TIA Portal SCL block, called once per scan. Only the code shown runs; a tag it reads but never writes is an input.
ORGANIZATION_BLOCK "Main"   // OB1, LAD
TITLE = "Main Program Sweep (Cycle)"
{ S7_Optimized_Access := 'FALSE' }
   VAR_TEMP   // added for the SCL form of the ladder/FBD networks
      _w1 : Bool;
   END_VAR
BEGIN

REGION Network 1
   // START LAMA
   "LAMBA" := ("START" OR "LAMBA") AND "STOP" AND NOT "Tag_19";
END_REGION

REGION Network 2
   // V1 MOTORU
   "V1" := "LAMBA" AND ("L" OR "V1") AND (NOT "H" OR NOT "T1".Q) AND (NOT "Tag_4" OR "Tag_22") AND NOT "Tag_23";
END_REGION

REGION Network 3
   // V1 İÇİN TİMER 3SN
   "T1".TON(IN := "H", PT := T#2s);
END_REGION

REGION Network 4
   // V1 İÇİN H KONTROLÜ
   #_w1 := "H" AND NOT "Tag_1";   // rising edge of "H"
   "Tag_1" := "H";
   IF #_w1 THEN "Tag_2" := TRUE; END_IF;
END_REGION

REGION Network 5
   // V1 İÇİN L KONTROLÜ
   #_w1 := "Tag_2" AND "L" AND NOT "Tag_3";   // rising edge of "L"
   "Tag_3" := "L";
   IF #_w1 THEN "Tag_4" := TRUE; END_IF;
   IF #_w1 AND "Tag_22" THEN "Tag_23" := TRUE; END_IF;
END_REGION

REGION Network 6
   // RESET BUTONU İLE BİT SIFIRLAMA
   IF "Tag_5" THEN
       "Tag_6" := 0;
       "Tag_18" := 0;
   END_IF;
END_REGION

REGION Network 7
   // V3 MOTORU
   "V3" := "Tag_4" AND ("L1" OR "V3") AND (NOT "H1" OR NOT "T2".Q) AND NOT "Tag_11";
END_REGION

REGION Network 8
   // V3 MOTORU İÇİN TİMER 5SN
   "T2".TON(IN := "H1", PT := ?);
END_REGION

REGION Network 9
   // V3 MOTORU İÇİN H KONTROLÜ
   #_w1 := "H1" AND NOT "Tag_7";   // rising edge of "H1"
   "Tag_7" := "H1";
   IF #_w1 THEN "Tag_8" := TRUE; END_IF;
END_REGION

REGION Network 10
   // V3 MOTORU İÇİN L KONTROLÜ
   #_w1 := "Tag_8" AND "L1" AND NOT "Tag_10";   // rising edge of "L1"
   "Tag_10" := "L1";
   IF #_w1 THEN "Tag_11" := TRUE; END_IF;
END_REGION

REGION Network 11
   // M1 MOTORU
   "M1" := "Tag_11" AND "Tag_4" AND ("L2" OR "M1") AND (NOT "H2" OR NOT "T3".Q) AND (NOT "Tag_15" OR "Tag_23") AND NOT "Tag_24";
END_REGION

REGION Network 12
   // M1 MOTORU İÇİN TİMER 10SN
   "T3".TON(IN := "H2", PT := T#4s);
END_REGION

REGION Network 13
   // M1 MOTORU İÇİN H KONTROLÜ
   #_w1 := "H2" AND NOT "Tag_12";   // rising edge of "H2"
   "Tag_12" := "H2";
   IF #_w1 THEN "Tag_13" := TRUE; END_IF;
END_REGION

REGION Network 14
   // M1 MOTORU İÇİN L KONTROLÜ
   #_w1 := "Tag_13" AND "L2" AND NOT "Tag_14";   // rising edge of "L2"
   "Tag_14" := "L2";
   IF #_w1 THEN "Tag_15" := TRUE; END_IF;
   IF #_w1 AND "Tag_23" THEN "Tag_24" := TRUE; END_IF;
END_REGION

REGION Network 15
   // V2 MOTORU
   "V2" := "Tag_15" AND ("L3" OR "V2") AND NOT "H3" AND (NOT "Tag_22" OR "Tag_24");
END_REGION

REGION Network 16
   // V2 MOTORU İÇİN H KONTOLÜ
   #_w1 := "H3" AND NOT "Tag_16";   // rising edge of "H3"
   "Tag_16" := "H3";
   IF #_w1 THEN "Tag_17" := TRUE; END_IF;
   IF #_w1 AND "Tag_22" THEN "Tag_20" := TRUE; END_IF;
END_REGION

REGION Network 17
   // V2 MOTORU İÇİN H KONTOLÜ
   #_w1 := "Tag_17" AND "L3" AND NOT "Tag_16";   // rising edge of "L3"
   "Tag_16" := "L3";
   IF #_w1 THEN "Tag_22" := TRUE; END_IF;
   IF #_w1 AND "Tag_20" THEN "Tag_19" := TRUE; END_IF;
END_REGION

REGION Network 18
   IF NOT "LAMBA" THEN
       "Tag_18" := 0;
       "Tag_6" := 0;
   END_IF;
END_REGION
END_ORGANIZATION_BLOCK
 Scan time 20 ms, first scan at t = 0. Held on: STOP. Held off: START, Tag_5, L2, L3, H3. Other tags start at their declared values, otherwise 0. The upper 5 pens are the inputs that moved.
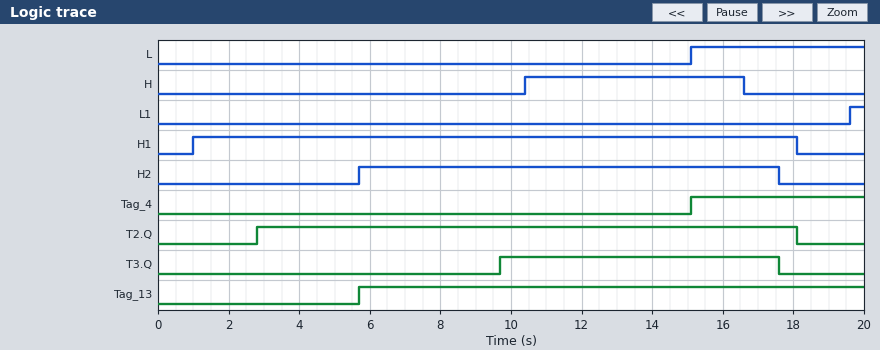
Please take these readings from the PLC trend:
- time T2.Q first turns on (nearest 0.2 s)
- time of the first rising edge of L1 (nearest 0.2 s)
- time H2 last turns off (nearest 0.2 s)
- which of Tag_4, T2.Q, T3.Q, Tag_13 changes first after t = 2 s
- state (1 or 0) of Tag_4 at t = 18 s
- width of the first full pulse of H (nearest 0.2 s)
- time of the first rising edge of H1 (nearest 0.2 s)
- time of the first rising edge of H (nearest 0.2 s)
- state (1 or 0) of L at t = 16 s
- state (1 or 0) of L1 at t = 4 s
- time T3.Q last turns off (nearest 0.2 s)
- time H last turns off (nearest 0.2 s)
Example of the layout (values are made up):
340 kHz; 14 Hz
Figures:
2.8 s; 19.6 s; 17.6 s; T2.Q; 1; 6.2 s; 1.0 s; 10.4 s; 1; 0; 17.6 s; 16.6 s
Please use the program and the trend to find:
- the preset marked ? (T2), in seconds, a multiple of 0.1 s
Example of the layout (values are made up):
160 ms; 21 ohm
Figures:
1.8 s
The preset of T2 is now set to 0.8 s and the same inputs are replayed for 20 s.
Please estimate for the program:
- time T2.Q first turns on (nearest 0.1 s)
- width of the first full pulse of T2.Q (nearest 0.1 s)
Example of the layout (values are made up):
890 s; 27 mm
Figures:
1.8 s; 16.3 s
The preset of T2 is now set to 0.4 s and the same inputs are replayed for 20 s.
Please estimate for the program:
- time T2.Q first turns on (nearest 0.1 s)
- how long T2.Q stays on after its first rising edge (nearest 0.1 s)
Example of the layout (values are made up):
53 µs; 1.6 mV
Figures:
1.4 s; 16.7 s
